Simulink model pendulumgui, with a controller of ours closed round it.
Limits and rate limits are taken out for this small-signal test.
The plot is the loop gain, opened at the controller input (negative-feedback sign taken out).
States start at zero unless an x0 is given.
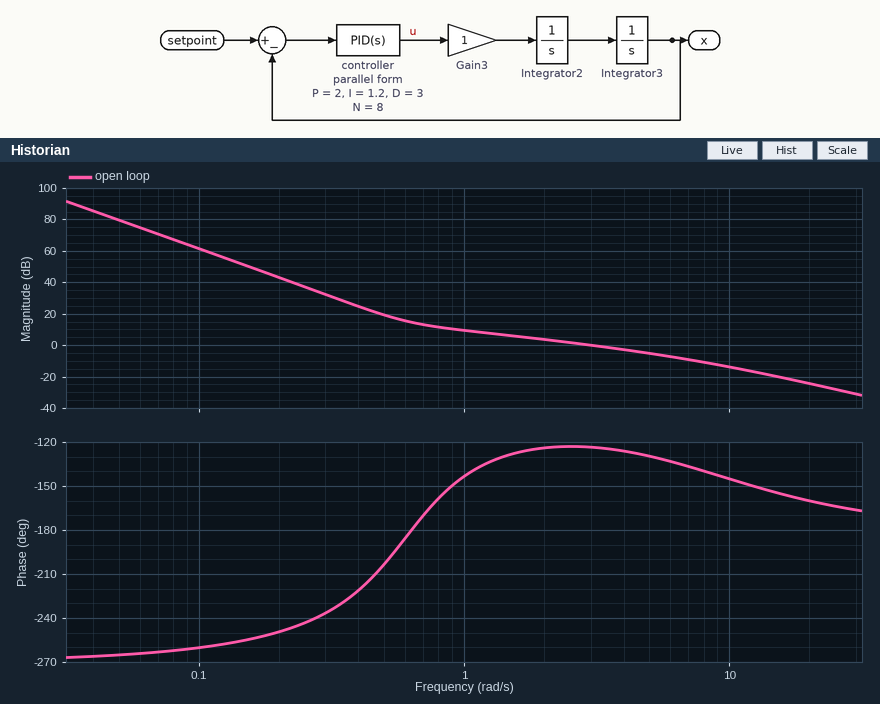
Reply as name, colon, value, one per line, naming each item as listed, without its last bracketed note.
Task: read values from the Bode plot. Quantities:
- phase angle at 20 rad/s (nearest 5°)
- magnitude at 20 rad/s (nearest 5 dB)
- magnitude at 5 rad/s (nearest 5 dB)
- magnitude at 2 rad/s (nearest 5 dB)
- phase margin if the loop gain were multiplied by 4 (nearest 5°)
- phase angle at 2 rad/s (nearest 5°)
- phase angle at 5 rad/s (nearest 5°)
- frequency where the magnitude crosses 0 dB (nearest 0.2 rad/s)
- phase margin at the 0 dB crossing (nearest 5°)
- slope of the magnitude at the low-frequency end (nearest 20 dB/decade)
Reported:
phase angle at 20 rad/s: -160°
magnitude at 20 rad/s: -25 dB
magnitude at 5 rad/s: -5 dB
magnitude at 2 rad/s: 5 dB
phase margin if the loop gain were multiplied by 4: 40°
phase angle at 2 rad/s: -125°
phase angle at 5 rad/s: -130°
frequency where the magnitude crosses 0 dB: 3.0 rad/s
phase margin at the 0 dB crossing: 55°
slope of the magnitude at the low-frequency end: -60 dB/decade
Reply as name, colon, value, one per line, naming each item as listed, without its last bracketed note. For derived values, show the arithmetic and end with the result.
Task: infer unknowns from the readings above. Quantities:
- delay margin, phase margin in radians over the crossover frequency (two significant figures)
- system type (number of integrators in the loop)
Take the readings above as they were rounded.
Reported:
delay margin, phase margin in radians over the crossover frequency: 55 × π / 180 / 3 = 0.32 s
system type: 3
